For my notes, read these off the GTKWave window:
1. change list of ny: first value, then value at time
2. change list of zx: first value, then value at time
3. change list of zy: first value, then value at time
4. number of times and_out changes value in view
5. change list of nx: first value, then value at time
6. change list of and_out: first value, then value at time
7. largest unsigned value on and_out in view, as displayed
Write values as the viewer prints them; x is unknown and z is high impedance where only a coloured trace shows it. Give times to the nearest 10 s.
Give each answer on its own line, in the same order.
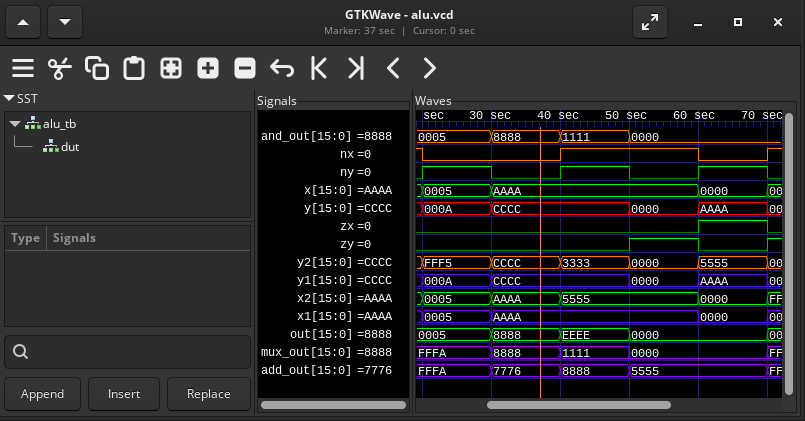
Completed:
0, 1 at 20 s, 0 at 30 s, 1 at 40 s, 0 at 50 s, 1 at 60 s, 0 at 70 s
0, 1 at 60 s, 0 at 70 s
0, 1 at 50 s, 0 at 60 s, 1 at 70 s
3
1, 0 at 20 s, 1 at 40 s, 0 at 60 s, 1 at 70 s
0005, 8888 at 30 s, 1111 at 40 s, 0000 at 50 s
8888
